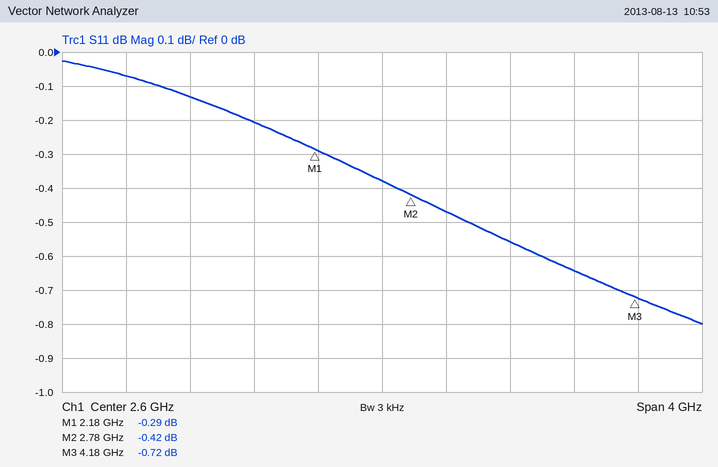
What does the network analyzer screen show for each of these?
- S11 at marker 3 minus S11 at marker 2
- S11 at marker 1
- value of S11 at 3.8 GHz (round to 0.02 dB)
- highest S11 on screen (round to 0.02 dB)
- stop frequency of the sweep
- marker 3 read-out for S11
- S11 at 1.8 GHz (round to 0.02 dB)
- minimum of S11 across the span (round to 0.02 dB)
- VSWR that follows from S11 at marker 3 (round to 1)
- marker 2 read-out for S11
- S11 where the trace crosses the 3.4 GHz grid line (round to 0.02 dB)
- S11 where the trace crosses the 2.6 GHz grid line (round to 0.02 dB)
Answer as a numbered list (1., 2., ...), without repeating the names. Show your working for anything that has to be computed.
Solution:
1. -0.72 − (-0.42) = -0.30 dB
2. -0.29 dB
3. -0.64 dB
4. -0.02 dB
5. 4.6 GHz
6. -0.72 dB
7. -0.20 dB
8. -0.80 dB
9. (1 + 0.9204)/(1 − 0.9204) ≈ 24
10. -0.42 dB
11. -0.56 dB
12. -0.38 dB
